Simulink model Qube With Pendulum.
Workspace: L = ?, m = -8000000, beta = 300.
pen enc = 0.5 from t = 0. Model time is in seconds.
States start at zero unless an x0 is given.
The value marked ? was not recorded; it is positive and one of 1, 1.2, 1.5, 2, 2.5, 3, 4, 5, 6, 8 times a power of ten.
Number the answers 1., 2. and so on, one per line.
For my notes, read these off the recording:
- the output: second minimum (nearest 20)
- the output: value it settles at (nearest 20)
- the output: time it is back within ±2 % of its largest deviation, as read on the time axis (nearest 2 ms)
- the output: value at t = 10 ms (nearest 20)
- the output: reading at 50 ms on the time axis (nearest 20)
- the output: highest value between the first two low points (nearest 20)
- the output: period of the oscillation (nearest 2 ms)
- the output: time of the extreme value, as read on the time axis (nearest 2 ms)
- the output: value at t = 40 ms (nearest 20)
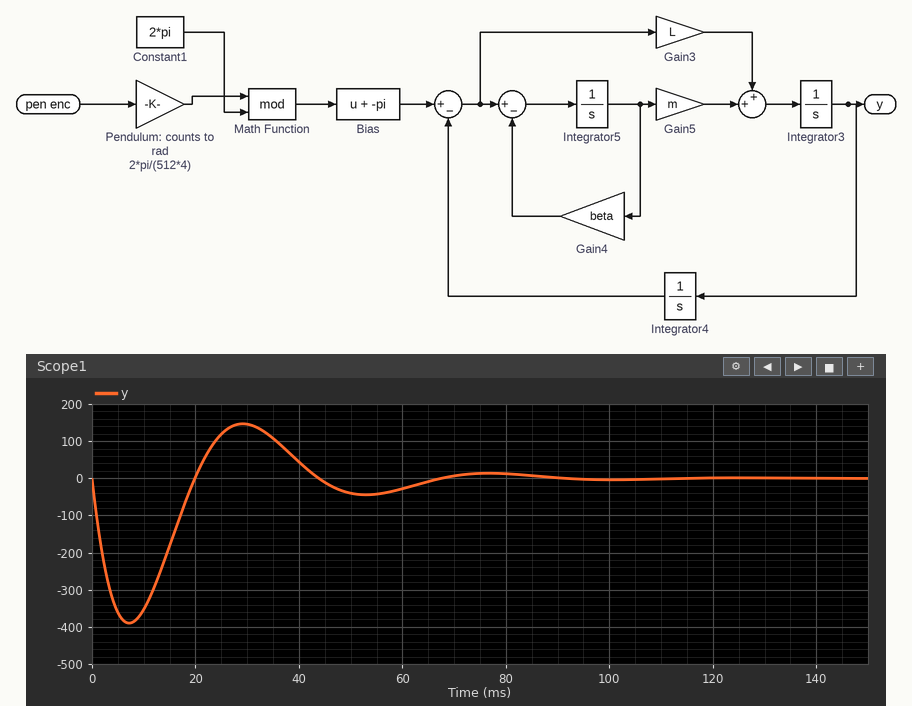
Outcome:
1. -40
2. 0
3. 84 ms
4. -360
5. -40
6. 140
7. 46 ms
8. 8 ms
9. 40
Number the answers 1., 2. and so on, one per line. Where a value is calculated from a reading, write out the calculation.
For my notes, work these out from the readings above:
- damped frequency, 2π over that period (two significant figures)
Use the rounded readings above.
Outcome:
1. 2π / 46 = 0.14 rad/ms
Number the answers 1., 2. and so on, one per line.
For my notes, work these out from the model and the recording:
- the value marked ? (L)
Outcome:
1. 40000
